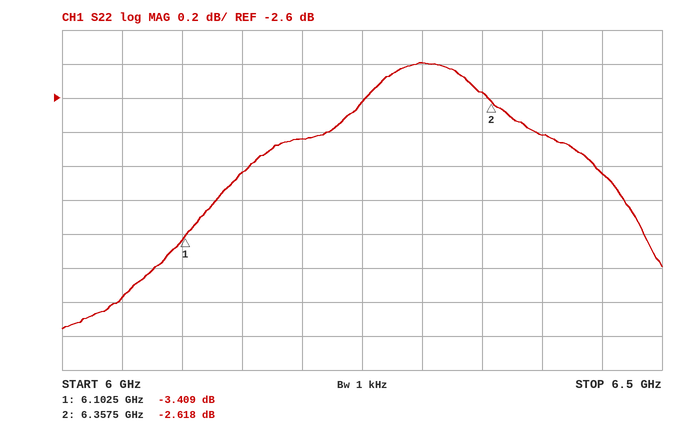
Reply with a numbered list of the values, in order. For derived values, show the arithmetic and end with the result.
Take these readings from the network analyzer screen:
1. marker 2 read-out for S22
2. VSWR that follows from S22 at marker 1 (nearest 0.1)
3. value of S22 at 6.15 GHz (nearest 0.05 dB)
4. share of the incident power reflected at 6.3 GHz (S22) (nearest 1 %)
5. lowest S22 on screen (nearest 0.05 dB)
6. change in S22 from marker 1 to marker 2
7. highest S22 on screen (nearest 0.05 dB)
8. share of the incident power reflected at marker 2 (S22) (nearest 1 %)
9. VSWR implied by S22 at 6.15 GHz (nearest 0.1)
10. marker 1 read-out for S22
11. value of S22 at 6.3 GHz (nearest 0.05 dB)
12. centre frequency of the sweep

1. -2.618 dB
2. (1 + 0.6754)/(1 − 0.6754) ≈ 5.2
3. -3.05 dB
4. 10^(-2.4/10) ≈ 58 %
5. -3.95 dB
6. -2.618 − (-3.409) = 0.791 dB
7. -2.40 dB
8. 10^(-2.618/10) ≈ 55 %
9. |Γ| = 10^(-3.05/20) = 0.7039; VSWR = (1 + 0.7039)/(1 − 0.7039) ≈ 5.8
10. -3.409 dB
11. -2.40 dB
12. 6.25 GHz
